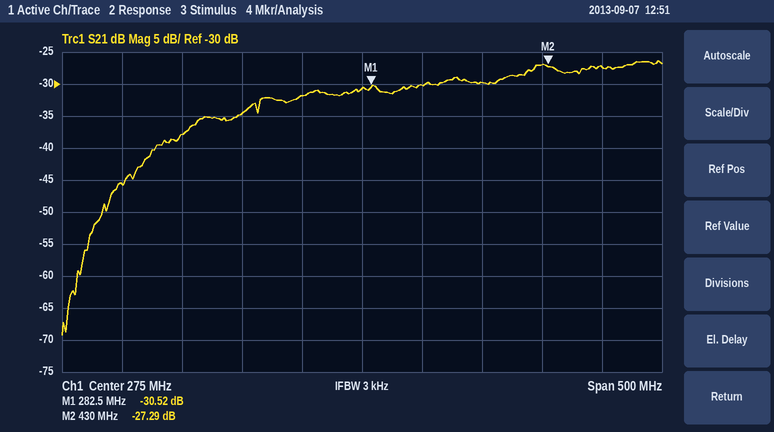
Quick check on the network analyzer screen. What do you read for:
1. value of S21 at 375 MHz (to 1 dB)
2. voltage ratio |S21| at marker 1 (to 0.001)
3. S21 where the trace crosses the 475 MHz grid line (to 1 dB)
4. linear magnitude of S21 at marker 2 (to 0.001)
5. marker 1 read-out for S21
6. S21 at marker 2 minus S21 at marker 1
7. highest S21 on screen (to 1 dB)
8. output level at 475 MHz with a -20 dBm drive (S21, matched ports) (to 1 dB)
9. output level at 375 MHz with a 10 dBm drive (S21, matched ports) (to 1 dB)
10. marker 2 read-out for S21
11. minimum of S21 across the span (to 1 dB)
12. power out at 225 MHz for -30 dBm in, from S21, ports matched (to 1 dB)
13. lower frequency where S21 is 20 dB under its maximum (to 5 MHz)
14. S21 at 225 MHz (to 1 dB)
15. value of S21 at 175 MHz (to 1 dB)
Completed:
-30 dB
0.030
-27 dB
0.043
-30.52 dB
3.23 dB
-26 dB
-47 dBm
-20 dBm
-27.29 dB
-69 dB
-62 dBm
70 MHz
-32 dB
-35 dB
